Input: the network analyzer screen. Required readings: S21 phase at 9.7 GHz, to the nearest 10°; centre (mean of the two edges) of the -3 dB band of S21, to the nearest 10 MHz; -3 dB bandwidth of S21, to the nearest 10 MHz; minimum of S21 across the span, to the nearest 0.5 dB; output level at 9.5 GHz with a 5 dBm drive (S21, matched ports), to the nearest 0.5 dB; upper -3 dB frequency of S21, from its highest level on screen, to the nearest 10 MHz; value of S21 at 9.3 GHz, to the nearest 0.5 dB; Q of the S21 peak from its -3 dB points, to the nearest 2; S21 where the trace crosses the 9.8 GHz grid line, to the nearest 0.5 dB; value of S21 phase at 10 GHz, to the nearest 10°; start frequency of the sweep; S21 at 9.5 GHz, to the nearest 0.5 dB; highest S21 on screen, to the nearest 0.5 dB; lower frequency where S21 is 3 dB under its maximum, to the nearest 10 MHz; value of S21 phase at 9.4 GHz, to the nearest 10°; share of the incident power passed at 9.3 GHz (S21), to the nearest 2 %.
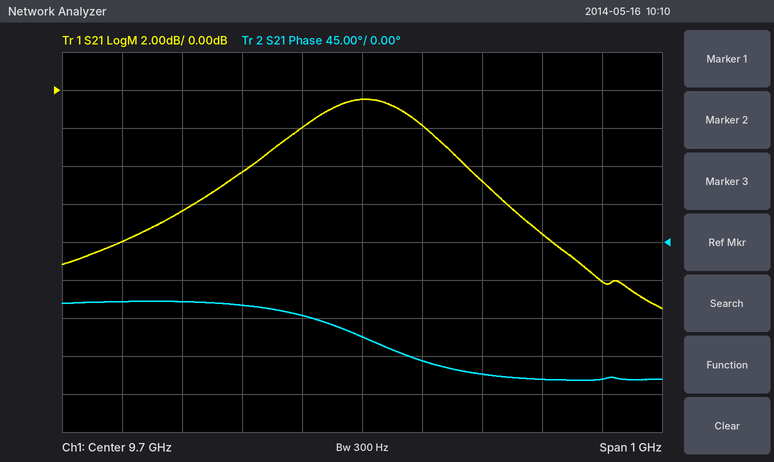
-110°
9.70 GHz
320 MHz
-11.5 dB
0.5 dBm
9.86 GHz
-8.0 dB
30
-2.0 dB
-160°
9.2 GHz
-4.5 dB
-0.5 dB
9.54 GHz
-70°
16 %
